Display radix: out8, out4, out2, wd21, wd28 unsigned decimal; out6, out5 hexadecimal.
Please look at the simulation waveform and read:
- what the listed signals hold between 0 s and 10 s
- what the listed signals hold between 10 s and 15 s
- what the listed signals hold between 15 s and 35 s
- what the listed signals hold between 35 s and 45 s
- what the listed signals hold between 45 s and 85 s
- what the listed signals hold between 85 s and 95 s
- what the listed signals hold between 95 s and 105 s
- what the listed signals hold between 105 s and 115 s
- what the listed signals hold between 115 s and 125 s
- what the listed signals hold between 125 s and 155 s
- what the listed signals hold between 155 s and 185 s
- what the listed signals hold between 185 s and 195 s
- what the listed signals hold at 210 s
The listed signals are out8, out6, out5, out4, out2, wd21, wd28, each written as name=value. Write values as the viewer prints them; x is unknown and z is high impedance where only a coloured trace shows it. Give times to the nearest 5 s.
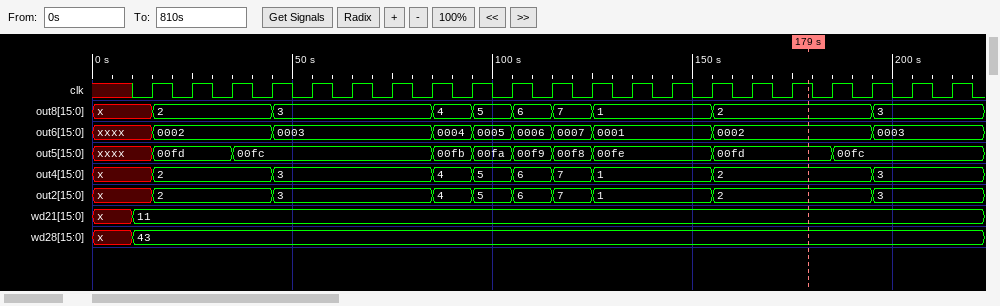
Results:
out8=x, out6=xxxx, out5=xxxx, out4=x, out2=x, wd21=x, wd28=x
out8=x, out6=xxxx, out5=xxxx, out4=x, out2=x, wd21=11, wd28=43
out8=2, out6=0002, out5=00fd, out4=2, out2=2, wd21=11, wd28=43
out8=2, out6=0002, out5=00fc, out4=2, out2=2, wd21=11, wd28=43
out8=3, out6=0003, out5=00fc, out4=3, out2=3, wd21=11, wd28=43
out8=4, out6=0004, out5=00fb, out4=4, out2=4, wd21=11, wd28=43
out8=5, out6=0005, out5=00fa, out4=5, out2=5, wd21=11, wd28=43
out8=6, out6=0006, out5=00f9, out4=6, out2=6, wd21=11, wd28=43
out8=7, out6=0007, out5=00f8, out4=7, out2=7, wd21=11, wd28=43
out8=1, out6=0001, out5=00fe, out4=1, out2=1, wd21=11, wd28=43
out8=2, out6=0002, out5=00fd, out4=2, out2=2, wd21=11, wd28=43
out8=2, out6=0002, out5=00fc, out4=2, out2=2, wd21=11, wd28=43
out8=3, out6=0003, out5=00fc, out4=3, out2=3, wd21=11, wd28=43
